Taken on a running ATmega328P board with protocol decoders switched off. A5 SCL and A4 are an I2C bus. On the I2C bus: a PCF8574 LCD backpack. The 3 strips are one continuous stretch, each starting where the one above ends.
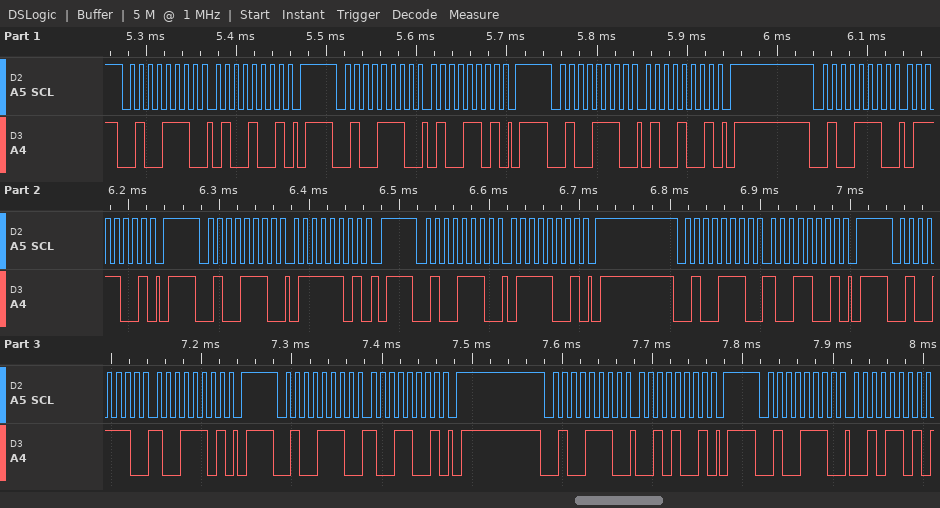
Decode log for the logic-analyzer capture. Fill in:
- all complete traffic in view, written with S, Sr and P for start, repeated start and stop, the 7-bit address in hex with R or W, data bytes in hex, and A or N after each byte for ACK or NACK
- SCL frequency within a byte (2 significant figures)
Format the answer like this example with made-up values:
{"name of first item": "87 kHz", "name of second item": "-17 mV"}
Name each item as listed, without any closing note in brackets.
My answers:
{"all complete traffic in view, written with S, Sr and P for start, repeated start and stop, the 7-bit address in hex with R or W, data bytes in hex, and A or N after each byte for ACK or NACK": "S 27W A 49 A P S 27W A 4D A P S 27W A 49 A P S 27W A 79 A P S 27W A 7D A P S 27W A 79 A P S 27W A 99 A P S 27W A 9D A P S 27W A 99 A P S 27W A 29 A P S 27W A 2D A", "SCL frequency within a byte": "100 kHz"}
